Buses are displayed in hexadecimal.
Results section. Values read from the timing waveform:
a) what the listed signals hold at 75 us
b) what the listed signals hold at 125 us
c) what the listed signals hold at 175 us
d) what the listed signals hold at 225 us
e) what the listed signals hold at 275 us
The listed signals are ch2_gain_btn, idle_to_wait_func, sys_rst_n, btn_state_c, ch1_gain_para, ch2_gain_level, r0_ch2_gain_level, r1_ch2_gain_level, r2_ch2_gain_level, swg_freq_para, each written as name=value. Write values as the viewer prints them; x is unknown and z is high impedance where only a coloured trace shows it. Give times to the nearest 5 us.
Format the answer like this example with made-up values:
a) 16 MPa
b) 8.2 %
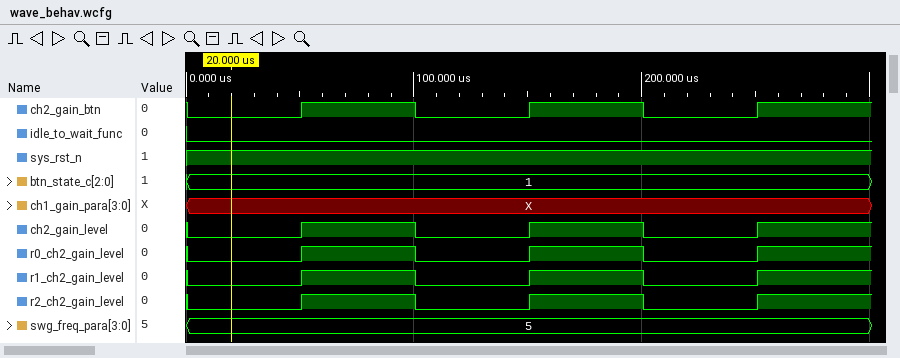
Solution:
a) ch2_gain_btn=1, idle_to_wait_func=0, sys_rst_n=1, btn_state_c=1, ch1_gain_para=X, ch2_gain_level=1, r0_ch2_gain_level=1, r1_ch2_gain_level=1, r2_ch2_gain_level=1, swg_freq_para=5
b) ch2_gain_btn=0, idle_to_wait_func=0, sys_rst_n=1, btn_state_c=1, ch1_gain_para=X, ch2_gain_level=0, r0_ch2_gain_level=0, r1_ch2_gain_level=0, r2_ch2_gain_level=0, swg_freq_para=5
c) ch2_gain_btn=1, idle_to_wait_func=0, sys_rst_n=1, btn_state_c=1, ch1_gain_para=X, ch2_gain_level=1, r0_ch2_gain_level=1, r1_ch2_gain_level=1, r2_ch2_gain_level=1, swg_freq_para=5
d) ch2_gain_btn=0, idle_to_wait_func=0, sys_rst_n=1, btn_state_c=1, ch1_gain_para=X, ch2_gain_level=0, r0_ch2_gain_level=0, r1_ch2_gain_level=0, r2_ch2_gain_level=0, swg_freq_para=5
e) ch2_gain_btn=1, idle_to_wait_func=0, sys_rst_n=1, btn_state_c=1, ch1_gain_para=X, ch2_gain_level=1, r0_ch2_gain_level=1, r1_ch2_gain_level=1, r2_ch2_gain_level=1, swg_freq_para=5
